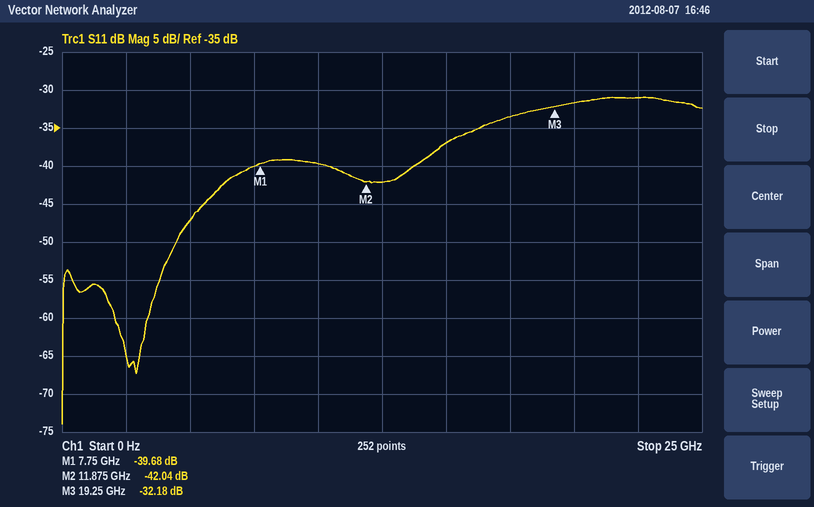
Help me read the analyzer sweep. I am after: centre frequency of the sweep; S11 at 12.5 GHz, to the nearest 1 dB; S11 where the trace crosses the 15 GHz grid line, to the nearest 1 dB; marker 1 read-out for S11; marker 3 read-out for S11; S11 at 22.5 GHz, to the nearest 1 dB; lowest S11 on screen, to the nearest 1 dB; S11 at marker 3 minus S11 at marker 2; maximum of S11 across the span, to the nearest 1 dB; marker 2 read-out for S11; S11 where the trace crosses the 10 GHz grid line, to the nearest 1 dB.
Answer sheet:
12.5 GHz
-42 dB
-37 dB
-39.68 dB
-32.18 dB
-31 dB
-74 dB
9.86 dB
-31 dB
-42.04 dB
-40 dB
